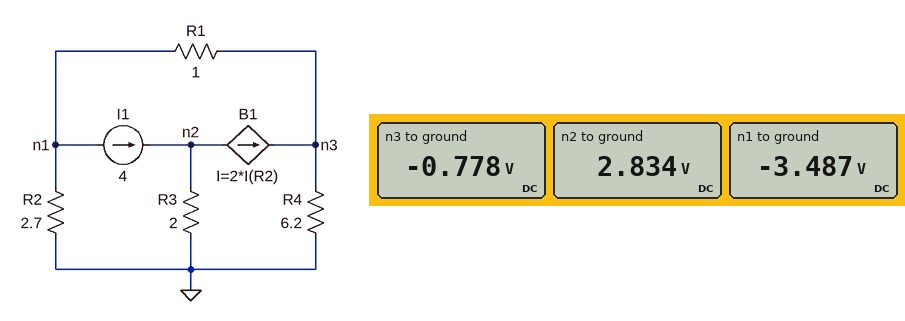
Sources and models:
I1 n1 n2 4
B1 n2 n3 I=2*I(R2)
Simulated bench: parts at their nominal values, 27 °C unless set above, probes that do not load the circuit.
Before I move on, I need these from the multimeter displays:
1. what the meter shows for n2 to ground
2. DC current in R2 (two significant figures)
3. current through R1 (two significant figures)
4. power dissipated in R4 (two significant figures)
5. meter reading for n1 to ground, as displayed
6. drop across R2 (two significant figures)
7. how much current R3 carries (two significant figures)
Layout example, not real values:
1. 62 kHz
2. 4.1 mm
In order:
1. 2.834 V
2. 1.3 A
3. 2.7 A
4. 98 mW
5. -3.487 V
6. 3.5 V
7. 1.4 A
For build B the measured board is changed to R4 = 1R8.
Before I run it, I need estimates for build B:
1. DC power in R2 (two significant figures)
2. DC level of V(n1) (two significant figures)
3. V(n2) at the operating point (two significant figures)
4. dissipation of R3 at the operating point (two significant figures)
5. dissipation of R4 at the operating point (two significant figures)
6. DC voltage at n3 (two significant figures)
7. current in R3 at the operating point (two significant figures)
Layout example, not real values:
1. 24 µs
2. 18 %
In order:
1. 4.1 W
2. -3.3 V
3. 3.1 V
4. 4.7 W
5. 170 mW
6. -550 mV
7. 1.5 A
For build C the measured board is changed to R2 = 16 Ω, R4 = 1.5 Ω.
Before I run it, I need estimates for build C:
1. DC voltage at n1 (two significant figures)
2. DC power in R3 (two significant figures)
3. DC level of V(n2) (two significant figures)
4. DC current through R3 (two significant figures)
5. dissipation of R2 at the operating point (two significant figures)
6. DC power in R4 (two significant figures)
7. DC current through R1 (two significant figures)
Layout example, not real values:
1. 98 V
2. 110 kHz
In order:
1. -7.4 V
2. 19 W
3. 6.1 V
4. 3.1 A
5. 3.5 W
6. 10 W
7. 3.5 A
